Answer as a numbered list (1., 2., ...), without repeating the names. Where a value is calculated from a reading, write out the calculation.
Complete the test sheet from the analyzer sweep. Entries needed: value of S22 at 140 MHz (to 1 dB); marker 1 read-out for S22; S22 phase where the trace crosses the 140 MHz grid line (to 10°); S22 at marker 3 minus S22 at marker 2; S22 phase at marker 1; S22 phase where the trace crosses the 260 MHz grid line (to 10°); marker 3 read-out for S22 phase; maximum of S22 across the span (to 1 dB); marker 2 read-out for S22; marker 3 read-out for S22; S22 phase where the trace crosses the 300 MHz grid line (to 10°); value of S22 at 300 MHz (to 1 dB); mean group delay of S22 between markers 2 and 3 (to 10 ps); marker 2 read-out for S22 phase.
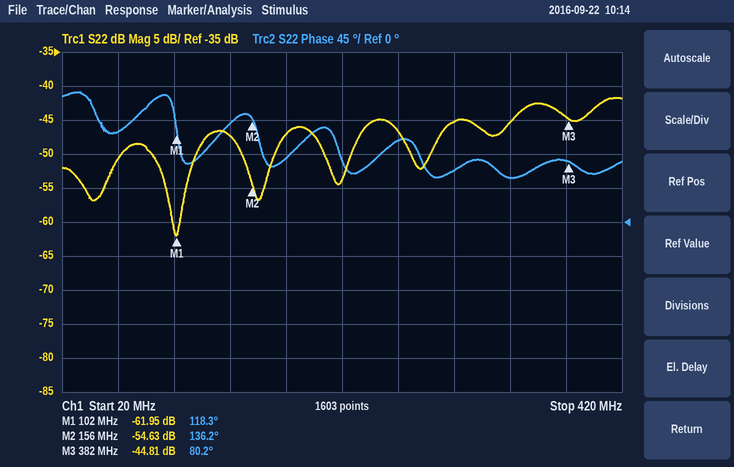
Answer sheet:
1. -47 dB
2. -61.95 dB
3. 130°
4. -44.81 − (-54.63) = 9.82 dB
5. 118.3°
6. 110°
7. 80.2°
8. -42 dB
9. -54.63 dB
10. -44.81 dB
11. 70°
12. -45 dB
13. −(80.2° − (136.2°))/(360° × 226 MHz) ≈ 688 ps, so 690 ps to the nearest 10 ps
14. 136.2°
